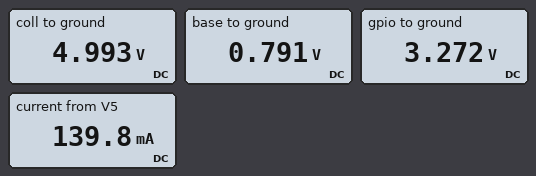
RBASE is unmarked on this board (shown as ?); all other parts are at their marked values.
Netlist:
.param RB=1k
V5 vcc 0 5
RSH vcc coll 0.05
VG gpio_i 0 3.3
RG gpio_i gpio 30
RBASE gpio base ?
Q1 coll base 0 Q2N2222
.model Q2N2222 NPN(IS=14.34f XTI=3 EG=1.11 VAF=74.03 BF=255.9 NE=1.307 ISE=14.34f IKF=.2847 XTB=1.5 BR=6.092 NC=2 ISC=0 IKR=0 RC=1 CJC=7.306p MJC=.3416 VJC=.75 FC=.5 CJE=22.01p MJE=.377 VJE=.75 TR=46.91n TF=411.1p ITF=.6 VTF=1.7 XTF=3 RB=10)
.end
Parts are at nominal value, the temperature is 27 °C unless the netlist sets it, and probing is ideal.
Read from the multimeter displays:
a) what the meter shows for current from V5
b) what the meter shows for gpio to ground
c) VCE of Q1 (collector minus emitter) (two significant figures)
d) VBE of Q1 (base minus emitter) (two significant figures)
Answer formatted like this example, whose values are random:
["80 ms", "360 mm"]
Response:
["139.8 mA", "3.272 V", "5.0 V", "790 mV"]
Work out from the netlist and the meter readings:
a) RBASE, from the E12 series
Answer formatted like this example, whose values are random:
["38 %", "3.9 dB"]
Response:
["2.7 kΩ"]
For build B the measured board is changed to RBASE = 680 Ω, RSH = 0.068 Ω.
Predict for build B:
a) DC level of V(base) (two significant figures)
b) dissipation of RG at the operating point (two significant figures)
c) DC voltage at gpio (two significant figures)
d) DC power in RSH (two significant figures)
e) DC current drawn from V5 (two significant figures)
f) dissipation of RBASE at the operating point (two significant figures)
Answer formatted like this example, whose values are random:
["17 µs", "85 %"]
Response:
["850 mV", "360 µW", "3.2 V", "9.0 mW", "360 mA", "8.1 mW"]
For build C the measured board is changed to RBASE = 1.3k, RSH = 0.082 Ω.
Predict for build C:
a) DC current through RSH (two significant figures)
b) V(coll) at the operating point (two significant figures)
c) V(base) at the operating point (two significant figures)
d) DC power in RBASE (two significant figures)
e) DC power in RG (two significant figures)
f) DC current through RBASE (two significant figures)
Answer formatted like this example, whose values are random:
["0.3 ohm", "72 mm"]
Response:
["240 mA", "5.0 V", "820 mV", "4.5 mW", "100 µW", "1.9 mA"]
